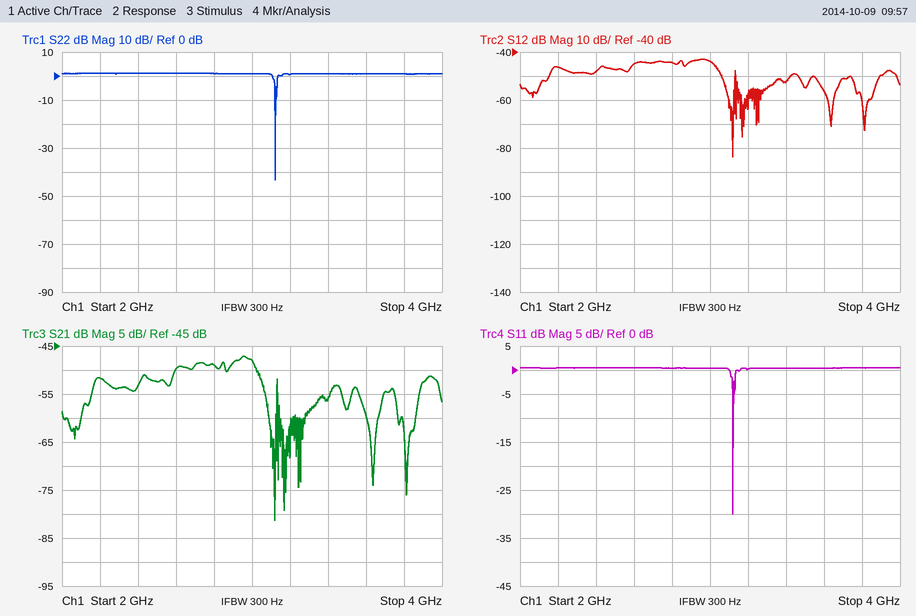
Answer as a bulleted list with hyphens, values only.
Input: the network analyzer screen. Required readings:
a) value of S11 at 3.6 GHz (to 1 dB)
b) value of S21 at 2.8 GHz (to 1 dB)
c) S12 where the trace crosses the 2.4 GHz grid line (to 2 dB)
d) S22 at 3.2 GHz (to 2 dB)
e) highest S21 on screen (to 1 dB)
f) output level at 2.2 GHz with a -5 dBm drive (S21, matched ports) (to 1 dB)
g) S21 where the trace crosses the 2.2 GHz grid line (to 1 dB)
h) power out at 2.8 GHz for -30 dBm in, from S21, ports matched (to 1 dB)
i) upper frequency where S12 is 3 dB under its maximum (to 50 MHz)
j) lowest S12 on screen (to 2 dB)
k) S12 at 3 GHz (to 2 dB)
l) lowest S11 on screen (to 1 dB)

- 0 dB
- -49 dB
- -48 dB
- 0 dB
- -47 dB
- -57 dBm
- -52 dB
- -79 dBm
- 3.05 GHz
- -84 dB
- -44 dB
- -30 dB
